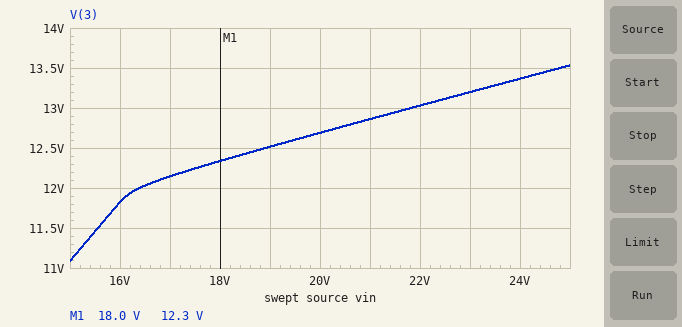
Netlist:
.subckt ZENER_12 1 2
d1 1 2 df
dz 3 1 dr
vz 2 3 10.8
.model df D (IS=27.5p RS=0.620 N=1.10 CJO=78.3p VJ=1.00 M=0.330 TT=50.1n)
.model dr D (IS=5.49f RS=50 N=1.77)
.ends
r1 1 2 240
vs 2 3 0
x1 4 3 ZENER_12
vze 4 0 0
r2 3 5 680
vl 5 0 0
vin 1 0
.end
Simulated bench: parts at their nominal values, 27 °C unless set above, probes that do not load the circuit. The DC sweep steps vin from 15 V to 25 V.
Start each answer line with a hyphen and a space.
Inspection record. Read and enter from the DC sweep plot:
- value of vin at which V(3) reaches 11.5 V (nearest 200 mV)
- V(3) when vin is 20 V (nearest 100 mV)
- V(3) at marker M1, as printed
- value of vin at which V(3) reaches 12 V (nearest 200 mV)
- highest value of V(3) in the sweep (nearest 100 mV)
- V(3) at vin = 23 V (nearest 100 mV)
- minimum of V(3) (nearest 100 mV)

- 15.6 V
- 12.7 V
- 12.3 V
- 16.4 V
- 13.5 V
- 13.2 V
- 11.1 V
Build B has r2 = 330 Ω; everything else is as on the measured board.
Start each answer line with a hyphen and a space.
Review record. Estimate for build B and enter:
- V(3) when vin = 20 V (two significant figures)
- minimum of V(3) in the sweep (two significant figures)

- 12 V
- 8.7 V
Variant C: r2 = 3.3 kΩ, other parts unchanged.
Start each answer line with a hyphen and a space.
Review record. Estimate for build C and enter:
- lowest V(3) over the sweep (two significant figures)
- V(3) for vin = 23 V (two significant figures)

- 12 V
- 14 V
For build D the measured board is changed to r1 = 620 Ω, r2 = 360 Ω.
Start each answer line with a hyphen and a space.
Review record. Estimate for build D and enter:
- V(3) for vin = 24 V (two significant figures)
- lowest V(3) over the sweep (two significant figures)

- 8.8 V
- 5.5 V
